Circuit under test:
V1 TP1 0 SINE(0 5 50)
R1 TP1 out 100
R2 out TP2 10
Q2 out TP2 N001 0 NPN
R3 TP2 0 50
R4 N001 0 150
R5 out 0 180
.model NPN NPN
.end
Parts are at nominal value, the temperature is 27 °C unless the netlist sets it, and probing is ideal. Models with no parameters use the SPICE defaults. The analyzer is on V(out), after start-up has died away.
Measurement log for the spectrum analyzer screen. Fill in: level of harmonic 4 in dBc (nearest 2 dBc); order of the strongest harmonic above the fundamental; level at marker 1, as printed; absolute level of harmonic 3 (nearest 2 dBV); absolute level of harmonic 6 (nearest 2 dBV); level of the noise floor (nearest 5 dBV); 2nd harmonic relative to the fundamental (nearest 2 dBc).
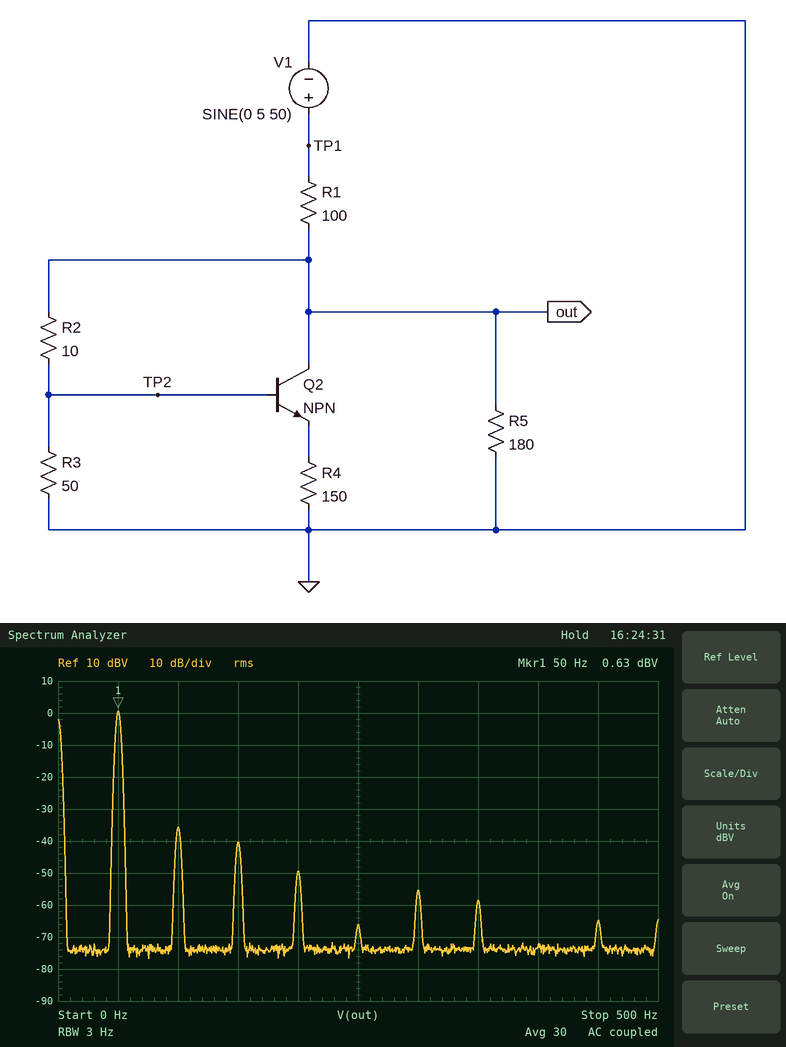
-50 dBc
2
0.63 dBV
-40 dBV
-56 dBV
-75 dBV
-36 dBc
